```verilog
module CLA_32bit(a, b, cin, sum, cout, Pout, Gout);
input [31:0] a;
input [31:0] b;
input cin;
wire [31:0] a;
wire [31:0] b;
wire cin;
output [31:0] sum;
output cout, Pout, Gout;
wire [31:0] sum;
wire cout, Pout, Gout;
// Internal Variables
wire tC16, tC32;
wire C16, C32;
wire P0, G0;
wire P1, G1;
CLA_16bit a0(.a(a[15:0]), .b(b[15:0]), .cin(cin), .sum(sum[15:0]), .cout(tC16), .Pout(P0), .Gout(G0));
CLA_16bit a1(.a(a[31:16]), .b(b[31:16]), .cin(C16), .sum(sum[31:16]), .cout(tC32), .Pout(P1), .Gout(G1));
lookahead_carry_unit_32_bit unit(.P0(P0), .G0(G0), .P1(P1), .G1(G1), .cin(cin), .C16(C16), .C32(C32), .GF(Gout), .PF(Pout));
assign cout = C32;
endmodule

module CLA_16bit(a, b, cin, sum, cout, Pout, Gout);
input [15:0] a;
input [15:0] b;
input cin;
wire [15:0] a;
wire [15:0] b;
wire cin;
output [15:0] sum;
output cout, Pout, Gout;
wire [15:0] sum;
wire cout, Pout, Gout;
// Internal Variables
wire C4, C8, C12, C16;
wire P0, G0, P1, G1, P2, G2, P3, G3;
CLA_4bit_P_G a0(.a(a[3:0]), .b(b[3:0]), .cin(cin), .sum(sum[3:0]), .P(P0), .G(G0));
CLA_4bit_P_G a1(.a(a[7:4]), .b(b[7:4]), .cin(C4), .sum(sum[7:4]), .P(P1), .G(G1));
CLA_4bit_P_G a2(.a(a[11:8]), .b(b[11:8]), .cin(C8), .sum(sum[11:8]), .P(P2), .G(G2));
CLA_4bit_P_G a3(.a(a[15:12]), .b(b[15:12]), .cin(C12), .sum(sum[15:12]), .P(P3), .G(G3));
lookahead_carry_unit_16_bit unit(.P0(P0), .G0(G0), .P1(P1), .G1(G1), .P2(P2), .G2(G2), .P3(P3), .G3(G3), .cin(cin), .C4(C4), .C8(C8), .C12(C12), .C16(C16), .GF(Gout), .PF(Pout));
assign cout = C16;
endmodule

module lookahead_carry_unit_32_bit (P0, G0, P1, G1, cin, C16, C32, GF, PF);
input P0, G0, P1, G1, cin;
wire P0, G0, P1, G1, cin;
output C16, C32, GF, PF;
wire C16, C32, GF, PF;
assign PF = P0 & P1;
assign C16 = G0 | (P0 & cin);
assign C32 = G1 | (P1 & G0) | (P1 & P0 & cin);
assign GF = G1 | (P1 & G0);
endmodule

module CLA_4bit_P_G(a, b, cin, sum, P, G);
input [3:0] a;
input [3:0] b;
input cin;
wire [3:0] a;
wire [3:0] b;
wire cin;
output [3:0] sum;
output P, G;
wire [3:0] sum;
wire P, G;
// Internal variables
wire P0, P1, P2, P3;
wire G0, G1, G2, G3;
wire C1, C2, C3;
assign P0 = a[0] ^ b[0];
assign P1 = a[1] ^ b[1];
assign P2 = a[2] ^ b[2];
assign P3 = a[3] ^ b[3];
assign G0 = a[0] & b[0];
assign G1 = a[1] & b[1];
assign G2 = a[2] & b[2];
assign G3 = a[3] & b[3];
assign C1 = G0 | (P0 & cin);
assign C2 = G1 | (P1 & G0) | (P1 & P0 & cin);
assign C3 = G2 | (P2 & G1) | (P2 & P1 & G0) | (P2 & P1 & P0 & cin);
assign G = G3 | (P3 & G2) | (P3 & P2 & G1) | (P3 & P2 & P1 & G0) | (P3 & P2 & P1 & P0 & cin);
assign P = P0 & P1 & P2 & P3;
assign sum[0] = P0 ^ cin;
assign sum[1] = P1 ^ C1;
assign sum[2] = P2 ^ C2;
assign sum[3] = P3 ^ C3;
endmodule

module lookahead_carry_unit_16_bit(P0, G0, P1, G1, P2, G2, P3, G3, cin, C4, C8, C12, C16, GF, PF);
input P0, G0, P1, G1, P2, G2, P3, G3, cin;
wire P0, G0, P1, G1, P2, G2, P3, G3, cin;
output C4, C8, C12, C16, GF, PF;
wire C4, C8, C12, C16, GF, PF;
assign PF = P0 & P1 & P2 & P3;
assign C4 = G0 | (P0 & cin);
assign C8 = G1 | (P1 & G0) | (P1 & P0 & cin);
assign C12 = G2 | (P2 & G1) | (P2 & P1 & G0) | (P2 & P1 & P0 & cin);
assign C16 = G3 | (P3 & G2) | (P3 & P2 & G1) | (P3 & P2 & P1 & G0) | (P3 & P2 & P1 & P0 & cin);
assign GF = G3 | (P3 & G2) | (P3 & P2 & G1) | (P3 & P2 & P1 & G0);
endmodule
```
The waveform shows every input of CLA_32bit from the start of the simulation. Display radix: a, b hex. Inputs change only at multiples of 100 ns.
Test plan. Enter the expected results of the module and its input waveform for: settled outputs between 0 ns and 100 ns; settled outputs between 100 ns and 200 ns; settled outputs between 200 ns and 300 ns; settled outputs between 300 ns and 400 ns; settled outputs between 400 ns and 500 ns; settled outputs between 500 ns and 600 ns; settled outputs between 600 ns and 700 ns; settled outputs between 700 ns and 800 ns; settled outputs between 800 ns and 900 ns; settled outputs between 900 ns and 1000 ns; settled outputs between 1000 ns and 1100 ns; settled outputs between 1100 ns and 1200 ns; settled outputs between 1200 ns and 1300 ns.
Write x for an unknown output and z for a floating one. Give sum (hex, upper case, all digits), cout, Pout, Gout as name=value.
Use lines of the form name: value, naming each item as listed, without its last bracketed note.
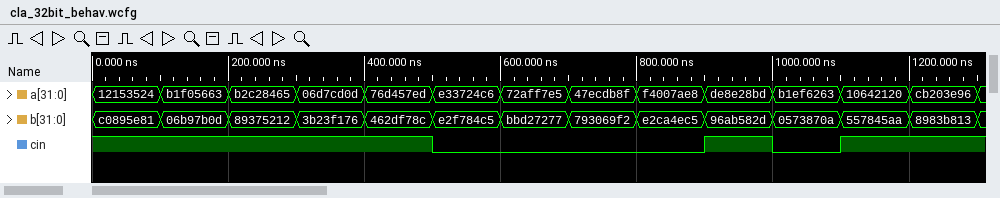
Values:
settled outputs between 0 ns and 100 ns: sum=D29E93A6, cout=0, Pout=0, Gout=0
settled outputs between 100 ns and 200 ns: sum=B8A9D171, cout=0, Pout=0, Gout=0
settled outputs between 200 ns and 300 ns: sum=3BF9D678, cout=1, Pout=0, Gout=1
settled outputs between 300 ns and 400 ns: sum=41FBBE84, cout=0, Pout=0, Gout=0
settled outputs between 400 ns and 500 ns: sum=BD024F7A, cout=0, Pout=0, Gout=0
settled outputs between 500 ns and 600 ns: sum=C62EA98B, cout=1, Pout=0, Gout=1
settled outputs between 600 ns and 700 ns: sum=2E826A5C, cout=1, Pout=0, Gout=1
settled outputs between 700 ns and 800 ns: sum=C11D4581, cout=0, Pout=0, Gout=0
settled outputs between 800 ns and 900 ns: sum=D6CAC9AD, cout=1, Pout=0, Gout=1
settled outputs between 900 ns and 1000 ns: sum=753980EB, cout=1, Pout=0, Gout=1
settled outputs between 1000 ns and 1100 ns: sum=B762E96D, cout=0, Pout=0, Gout=0
settled outputs between 1100 ns and 1200 ns: sum=65DC66CB, cout=0, Pout=0, Gout=0
settled outputs between 1200 ns and 1300 ns: sum=54A3F6AA, cout=1, Pout=0, Gout=1
